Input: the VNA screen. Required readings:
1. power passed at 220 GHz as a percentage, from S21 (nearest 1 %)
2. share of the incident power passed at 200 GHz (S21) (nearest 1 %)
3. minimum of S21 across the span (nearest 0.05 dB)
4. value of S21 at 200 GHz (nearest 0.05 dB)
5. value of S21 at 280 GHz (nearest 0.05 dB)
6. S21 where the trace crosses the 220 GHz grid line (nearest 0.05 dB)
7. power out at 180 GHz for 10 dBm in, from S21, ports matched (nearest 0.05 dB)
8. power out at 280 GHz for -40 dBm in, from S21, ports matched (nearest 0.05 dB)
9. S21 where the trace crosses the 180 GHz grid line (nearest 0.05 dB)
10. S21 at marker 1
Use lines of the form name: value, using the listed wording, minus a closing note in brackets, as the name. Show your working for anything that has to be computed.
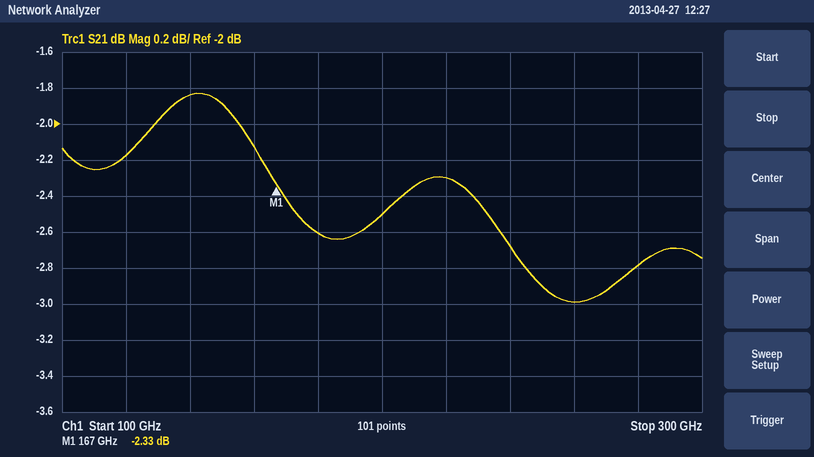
power passed at 220 GHz as a percentage, from S21: 10^(-2.3/10) ≈ 59 %
share of the incident power passed at 200 GHz (S21): 10^(-2.5/10) ≈ 56 %
minimum of S21 across the span: -3.00 dB
value of S21 at 200 GHz: -2.50 dB
value of S21 at 280 GHz: -2.80 dB
S21 where the trace crosses the 220 GHz grid line: -2.30 dB
power out at 180 GHz for 10 dBm in, from S21, ports matched: 10 dBm + (-2.60 dB) = 7.40 dBm
power out at 280 GHz for -40 dBm in, from S21, ports matched: -40 dBm + (-2.80 dB) = -42.80 dBm
S21 where the trace crosses the 180 GHz grid line: -2.60 dB
S21 at marker 1: -2.33 dB
